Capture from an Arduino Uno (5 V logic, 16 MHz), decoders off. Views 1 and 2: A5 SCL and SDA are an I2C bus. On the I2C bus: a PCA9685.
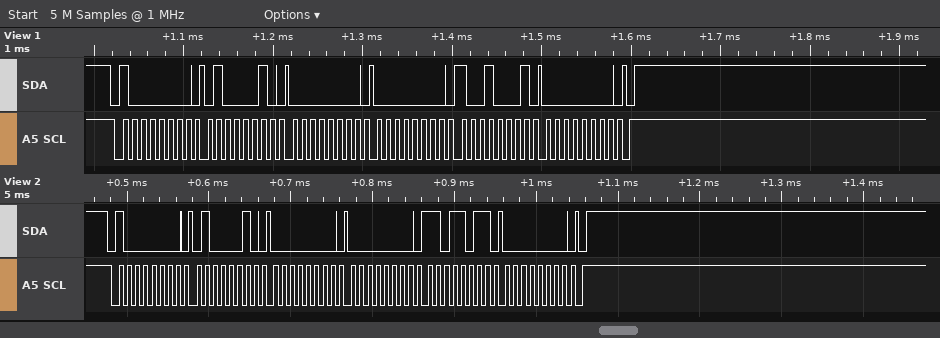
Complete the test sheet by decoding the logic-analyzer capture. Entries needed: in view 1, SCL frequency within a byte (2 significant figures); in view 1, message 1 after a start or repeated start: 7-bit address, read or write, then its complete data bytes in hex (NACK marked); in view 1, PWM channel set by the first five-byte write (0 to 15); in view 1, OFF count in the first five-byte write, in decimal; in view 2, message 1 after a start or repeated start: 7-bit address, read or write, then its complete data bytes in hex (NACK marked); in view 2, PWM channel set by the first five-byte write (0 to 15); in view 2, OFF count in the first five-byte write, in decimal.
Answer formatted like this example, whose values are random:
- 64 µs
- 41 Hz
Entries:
- 100 kHz
- 0x40 write: 42 00 00 91 00
- 15
- 145
- 0x40 write: 42 00 00 DB 00
- 15
- 219
